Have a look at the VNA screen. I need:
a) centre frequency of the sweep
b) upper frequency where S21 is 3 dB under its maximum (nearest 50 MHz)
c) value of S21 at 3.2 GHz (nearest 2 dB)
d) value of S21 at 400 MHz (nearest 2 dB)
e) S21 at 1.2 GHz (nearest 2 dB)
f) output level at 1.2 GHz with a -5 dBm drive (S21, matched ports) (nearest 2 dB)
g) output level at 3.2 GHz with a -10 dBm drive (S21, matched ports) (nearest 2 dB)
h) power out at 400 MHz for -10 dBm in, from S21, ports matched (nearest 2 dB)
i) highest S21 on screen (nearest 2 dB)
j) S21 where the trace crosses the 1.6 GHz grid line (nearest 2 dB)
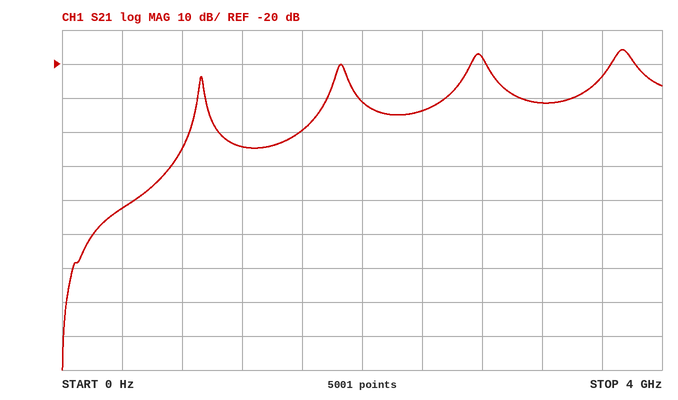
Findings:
2 GHz
3.80 GHz
-32 dB
-62 dB
-44 dB
-50 dBm
-42 dBm
-72 dBm
-16 dB
-40 dB
